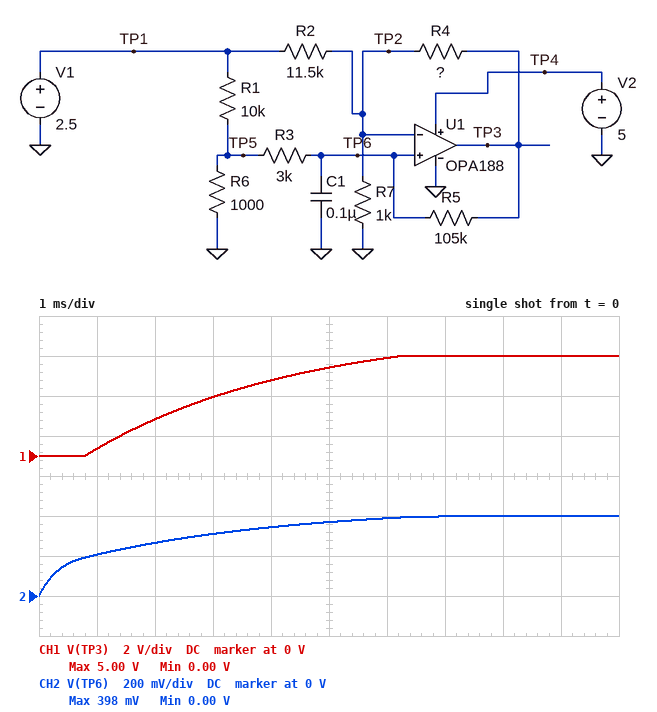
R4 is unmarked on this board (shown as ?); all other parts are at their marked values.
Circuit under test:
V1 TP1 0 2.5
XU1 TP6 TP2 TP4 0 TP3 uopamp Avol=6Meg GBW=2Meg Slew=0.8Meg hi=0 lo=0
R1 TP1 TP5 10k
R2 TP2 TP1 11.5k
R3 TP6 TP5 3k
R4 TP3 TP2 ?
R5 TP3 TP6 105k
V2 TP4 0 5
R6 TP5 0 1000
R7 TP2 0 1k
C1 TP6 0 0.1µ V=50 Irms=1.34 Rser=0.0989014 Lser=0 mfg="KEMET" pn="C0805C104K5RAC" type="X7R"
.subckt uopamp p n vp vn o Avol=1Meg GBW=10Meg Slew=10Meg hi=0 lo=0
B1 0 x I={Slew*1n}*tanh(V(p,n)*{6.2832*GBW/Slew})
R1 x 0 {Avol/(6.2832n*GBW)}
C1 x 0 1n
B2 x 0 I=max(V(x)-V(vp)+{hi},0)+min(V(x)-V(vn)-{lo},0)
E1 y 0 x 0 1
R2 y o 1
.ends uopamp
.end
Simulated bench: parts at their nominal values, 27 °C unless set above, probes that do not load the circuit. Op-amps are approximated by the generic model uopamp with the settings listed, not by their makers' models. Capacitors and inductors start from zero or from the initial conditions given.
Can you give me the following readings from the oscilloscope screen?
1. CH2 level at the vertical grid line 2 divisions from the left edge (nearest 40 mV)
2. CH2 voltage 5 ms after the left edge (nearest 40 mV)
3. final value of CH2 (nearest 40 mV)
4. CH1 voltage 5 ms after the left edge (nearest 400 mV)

280 mV
360 mV
400 mV
4.4 V
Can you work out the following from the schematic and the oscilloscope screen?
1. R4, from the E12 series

22 kΩ
